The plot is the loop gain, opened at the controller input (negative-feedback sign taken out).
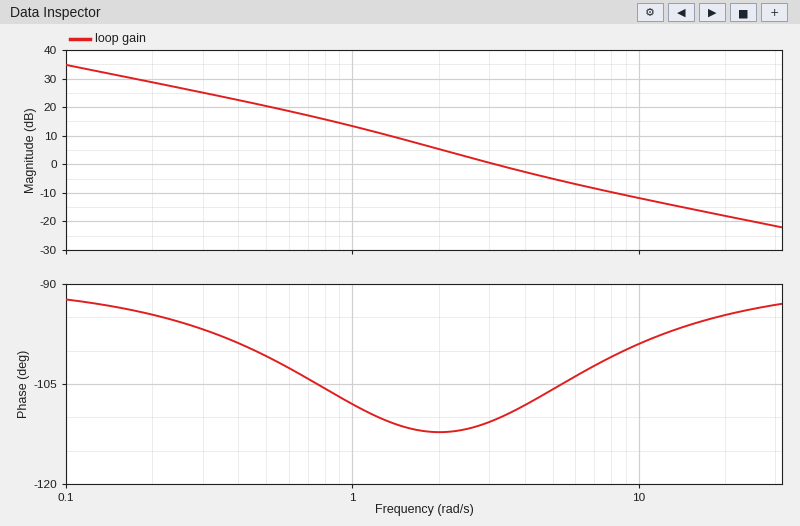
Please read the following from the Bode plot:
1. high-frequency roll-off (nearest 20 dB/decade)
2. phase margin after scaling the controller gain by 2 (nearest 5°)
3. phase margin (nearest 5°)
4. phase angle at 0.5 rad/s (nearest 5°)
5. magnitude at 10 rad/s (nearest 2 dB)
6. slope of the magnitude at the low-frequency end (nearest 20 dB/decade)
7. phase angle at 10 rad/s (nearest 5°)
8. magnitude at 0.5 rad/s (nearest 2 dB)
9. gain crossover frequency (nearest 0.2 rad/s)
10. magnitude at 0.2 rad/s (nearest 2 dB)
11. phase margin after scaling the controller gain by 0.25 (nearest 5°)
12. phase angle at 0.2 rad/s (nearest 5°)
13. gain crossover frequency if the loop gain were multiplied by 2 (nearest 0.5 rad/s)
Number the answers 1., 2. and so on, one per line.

1. -20 dB/decade
2. 75°
3. 70°
4. -100°
5. -12 dB
6. -20 dB/decade
7. -100°
8. 20 dB
9. 3.2 rad/s
10. 28 dB
11. 70°
12. -95°
13. 5.5 rad/s
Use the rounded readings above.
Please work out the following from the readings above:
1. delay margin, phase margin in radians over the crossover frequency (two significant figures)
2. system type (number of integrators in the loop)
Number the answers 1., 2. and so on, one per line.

1. 0.38 s
2. 1
